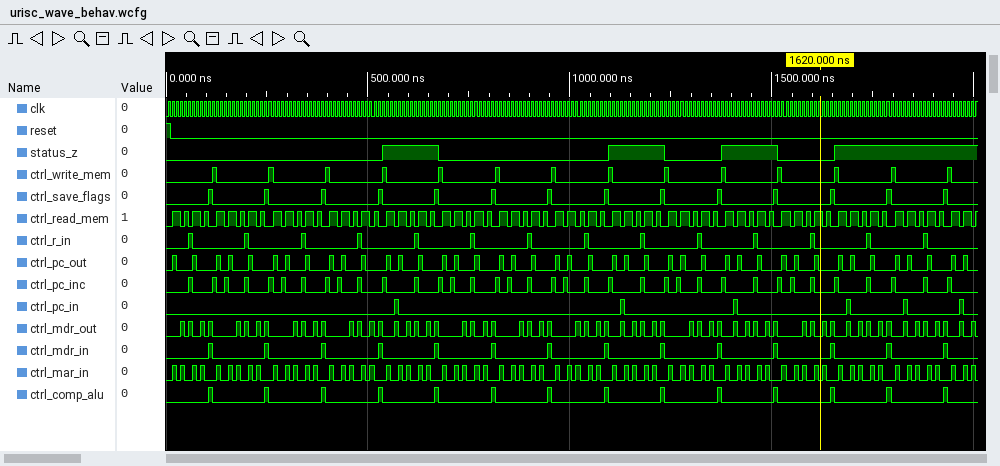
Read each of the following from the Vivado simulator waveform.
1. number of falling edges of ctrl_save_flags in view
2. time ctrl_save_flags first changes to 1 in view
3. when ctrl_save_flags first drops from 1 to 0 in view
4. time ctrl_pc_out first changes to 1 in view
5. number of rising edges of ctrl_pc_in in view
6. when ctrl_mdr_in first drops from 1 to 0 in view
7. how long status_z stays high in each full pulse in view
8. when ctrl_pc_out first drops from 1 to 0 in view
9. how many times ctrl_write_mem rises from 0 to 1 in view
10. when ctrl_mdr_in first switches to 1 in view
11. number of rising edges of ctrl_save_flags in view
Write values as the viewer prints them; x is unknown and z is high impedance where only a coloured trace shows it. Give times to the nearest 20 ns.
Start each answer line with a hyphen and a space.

- 14
- 100 ns
- 120 ns
- 20 ns
- 6
- 120 ns
- 140 ns, 140 ns, 140 ns
- 20 ns
- 14
- 100 ns
- 14
